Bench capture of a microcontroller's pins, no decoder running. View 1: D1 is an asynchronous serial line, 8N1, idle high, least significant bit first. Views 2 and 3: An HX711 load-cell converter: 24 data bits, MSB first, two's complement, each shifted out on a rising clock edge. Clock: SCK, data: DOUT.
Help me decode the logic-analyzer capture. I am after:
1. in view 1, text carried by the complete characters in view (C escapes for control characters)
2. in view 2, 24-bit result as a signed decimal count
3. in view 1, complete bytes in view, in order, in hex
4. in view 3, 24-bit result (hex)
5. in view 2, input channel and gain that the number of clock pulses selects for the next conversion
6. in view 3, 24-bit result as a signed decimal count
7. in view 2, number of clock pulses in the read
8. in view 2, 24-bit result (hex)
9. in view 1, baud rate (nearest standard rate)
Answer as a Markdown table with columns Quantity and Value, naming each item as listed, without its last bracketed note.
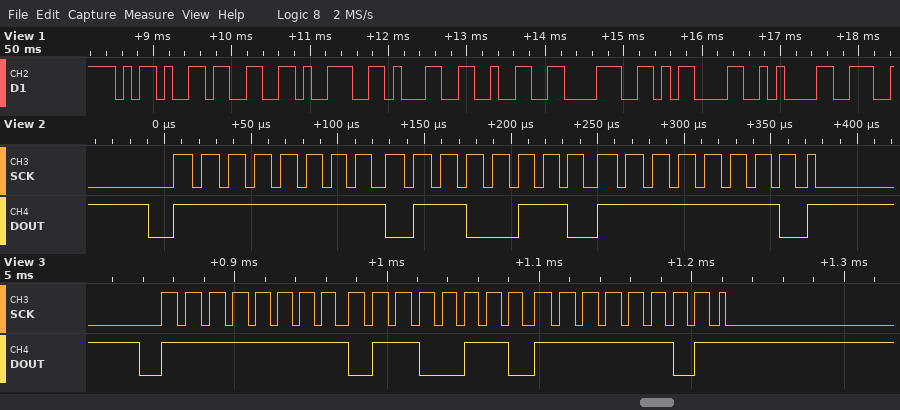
| Quantity | Value |
|---|---|
| in view 1, text carried by the complete characters in view | "-39128\r\n" |
| in view 2, 24-bit result as a signed decimal count | -39170 |
| in view 1, complete bytes in view, in order, in hex | 2D 33 39 31 32 38 0D 0A |
| in view 3, 24-bit result | 0xFF66FD |
| in view 2, input channel and gain that the number of clock pulses selects for the next conversion | channel A, gain 128 |
| in view 3, 24-bit result as a signed decimal count | -39171 |
| in view 2, number of clock pulses in the read | 25 |
| in view 2, 24-bit result | 0xFF66FE |
| in view 1, baud rate | 9600 baud |
